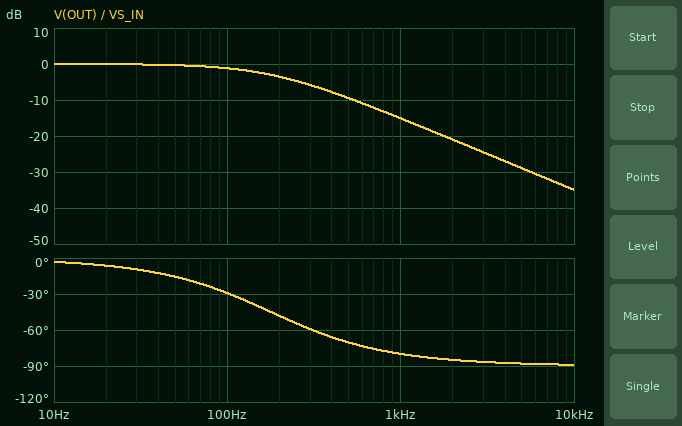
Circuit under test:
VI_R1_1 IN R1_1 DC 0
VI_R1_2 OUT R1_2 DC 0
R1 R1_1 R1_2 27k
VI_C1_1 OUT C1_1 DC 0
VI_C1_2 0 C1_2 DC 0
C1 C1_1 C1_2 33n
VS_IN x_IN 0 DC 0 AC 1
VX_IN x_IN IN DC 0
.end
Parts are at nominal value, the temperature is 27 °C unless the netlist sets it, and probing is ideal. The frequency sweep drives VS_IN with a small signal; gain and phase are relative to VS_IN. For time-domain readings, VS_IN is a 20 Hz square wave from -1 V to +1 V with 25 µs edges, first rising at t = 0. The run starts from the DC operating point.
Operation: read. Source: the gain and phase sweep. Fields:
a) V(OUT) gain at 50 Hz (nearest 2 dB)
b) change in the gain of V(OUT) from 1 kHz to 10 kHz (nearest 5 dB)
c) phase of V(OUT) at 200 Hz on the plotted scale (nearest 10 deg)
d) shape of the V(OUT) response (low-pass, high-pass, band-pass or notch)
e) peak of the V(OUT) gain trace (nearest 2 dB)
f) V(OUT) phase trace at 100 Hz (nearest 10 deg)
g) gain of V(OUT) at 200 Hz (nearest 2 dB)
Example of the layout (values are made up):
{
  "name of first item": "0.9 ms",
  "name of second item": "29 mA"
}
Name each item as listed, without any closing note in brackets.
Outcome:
{
  "V(OUT) gain at 50 Hz": "0 dB",
  "change in the gain of V(OUT) from 1 kHz to 10 kHz": "-20 dB",
  "phase of V(OUT) at 200 Hz on the plotted scale": "-50 deg",
  "shape of the V(OUT) response": "low-pass",
  "peak of the V(OUT) gain trace": "0 dB",
  "V(OUT) phase trace at 100 Hz": "-30 deg",
  "gain of V(OUT) at 200 Hz": "-4 dB"
}
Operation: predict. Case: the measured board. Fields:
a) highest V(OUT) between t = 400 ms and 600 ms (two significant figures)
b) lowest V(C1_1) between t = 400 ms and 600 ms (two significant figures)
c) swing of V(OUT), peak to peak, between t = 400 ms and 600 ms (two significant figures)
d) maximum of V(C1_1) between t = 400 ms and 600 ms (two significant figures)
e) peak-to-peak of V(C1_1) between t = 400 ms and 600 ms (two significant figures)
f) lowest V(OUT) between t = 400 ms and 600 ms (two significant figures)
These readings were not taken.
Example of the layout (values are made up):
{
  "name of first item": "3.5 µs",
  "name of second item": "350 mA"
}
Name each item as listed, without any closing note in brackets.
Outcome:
{
  "highest V(OUT) between t = 400 ms and 600 ms": "1.0 V",
  "lowest V(C1_1) between t = 400 ms and 600 ms": "-1.0 V",
  "swing of V(OUT), peak to peak, between t = 400 ms and 600 ms": "2.0 V",
  "maximum of V(C1_1) between t = 400 ms and 600 ms": "1.0 V",
  "peak-to-peak of V(C1_1) between t = 400 ms and 600 ms": "2.0 V",
  "lowest V(OUT) between t = 400 ms and 600 ms": "-1.0 V"
}
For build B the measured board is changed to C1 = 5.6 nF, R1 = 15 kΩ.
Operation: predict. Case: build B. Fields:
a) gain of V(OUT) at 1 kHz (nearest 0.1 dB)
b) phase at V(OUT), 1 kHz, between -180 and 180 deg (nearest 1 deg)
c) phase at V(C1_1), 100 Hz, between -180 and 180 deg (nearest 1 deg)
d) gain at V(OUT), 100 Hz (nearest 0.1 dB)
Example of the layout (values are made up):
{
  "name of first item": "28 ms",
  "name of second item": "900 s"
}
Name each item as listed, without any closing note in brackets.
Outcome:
{
  "gain of V(OUT) at 1 kHz": "-1.1 dB",
  "phase at V(OUT), 1 kHz, between -180 and 180 deg": "-28 deg",
  "phase at V(C1_1), 100 Hz, between -180 and 180 deg": "-3 deg",
  "gain at V(OUT), 100 Hz": "0 dB"
}
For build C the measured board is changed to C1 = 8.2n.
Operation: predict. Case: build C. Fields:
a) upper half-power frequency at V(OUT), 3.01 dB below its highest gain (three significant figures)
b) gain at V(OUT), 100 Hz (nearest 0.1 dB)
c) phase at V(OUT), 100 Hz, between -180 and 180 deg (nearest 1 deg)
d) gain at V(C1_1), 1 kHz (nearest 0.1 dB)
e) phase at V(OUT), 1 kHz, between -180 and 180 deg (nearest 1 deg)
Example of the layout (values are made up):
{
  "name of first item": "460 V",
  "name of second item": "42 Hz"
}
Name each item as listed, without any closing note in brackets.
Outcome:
{
  "upper half-power frequency at V(OUT), 3.01 dB below its highest gain": "719 Hz",
  "gain at V(OUT), 100 Hz": "-0.1 dB",
  "phase at V(OUT), 100 Hz, between -180 and 180 deg": "-8 deg",
  "gain at V(C1_1), 1 kHz": "-4.7 dB",
  "phase at V(OUT), 1 kHz, between -180 and 180 deg": "-54 deg"
}
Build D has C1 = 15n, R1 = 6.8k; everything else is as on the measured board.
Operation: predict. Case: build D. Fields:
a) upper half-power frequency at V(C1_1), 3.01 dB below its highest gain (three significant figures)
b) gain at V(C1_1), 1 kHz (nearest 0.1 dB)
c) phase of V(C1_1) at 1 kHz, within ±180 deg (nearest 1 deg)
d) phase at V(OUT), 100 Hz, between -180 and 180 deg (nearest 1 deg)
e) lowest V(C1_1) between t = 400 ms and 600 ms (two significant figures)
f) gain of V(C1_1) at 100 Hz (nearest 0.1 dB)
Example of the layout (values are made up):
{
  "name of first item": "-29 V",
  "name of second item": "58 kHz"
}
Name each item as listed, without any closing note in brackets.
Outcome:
{
  "upper half-power frequency at V(C1_1), 3.01 dB below its highest gain": "1.56 kHz",
  "gain at V(C1_1), 1 kHz": "-1.5 dB",
  "phase of V(C1_1) at 1 kHz, within ±180 deg": "-33 deg",
  "phase at V(OUT), 100 Hz, between -180 and 180 deg": "-4 deg",
  "lowest V(C1_1) between t = 400 ms and 600 ms": "-1.0 V",
  "gain of V(C1_1) at 100 Hz": "0 dB"
}
